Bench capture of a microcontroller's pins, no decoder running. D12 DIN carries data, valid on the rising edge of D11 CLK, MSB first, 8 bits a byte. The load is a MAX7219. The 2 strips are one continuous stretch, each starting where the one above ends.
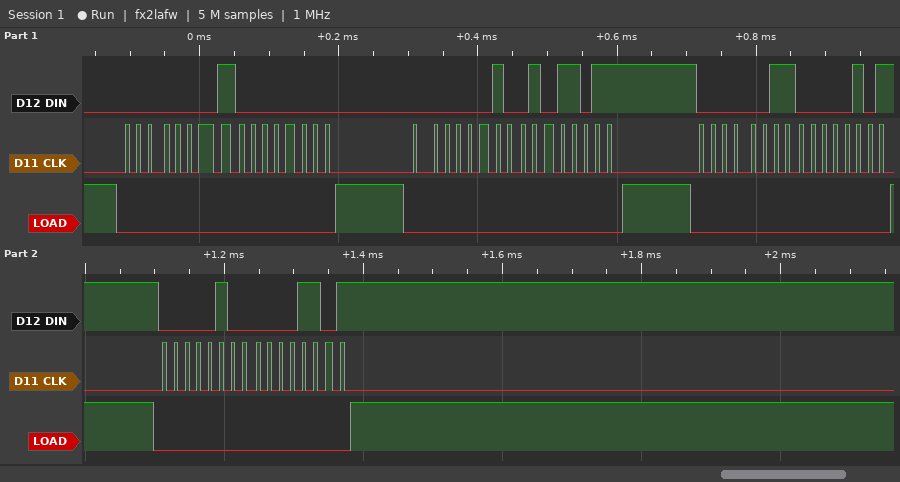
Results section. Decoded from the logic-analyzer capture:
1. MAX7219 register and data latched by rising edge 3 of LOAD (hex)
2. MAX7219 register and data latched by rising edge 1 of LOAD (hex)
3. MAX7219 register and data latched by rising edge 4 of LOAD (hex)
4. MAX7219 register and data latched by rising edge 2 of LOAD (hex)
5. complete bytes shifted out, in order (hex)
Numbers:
register 0x3, data 0x05
register 0x1, data 0x00
register 0x4, data 0x0D
register 0x2, data 0x5B
01 00 02 5B 03 05 04 0D
